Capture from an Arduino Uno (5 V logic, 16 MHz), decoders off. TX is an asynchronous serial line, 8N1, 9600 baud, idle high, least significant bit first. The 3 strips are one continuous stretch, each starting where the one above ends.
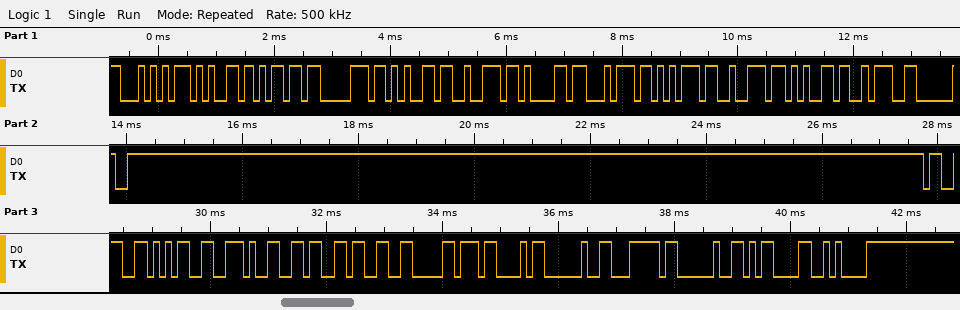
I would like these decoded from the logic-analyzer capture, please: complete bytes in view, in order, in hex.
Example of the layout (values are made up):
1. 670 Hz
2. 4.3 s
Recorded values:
1. 0x54 0x65 0x6D 0x70 0x65 0x72 0x61 0x74 0x75 0x72 0x65 0x3A 0x20 0x33 0x35 0x2E 0x36 0x33 0xB0 0x43 0x20 0x7C 0x20 0x0D 0x0A
